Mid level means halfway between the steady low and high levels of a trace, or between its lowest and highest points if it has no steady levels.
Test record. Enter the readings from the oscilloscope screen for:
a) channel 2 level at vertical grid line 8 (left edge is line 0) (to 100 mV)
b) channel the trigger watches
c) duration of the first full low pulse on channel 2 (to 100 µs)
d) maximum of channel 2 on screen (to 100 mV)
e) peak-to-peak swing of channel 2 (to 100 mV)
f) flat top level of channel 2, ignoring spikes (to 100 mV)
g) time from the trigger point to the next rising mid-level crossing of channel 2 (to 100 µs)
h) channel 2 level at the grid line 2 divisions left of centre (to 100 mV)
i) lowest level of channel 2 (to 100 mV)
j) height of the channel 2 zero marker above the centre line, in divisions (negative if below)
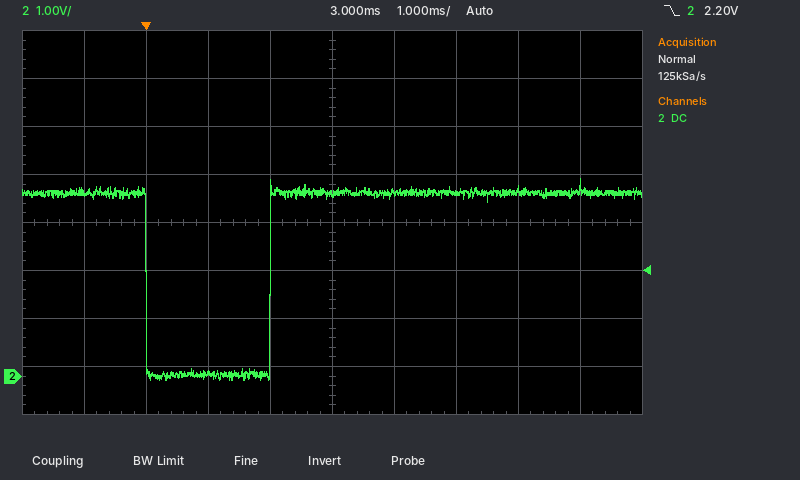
3.9 V
channel 2
2.0 ms
4.1 V
4.2 V
3.8 V
2.0 ms
100 mV
-100 mV
-3.2 div
